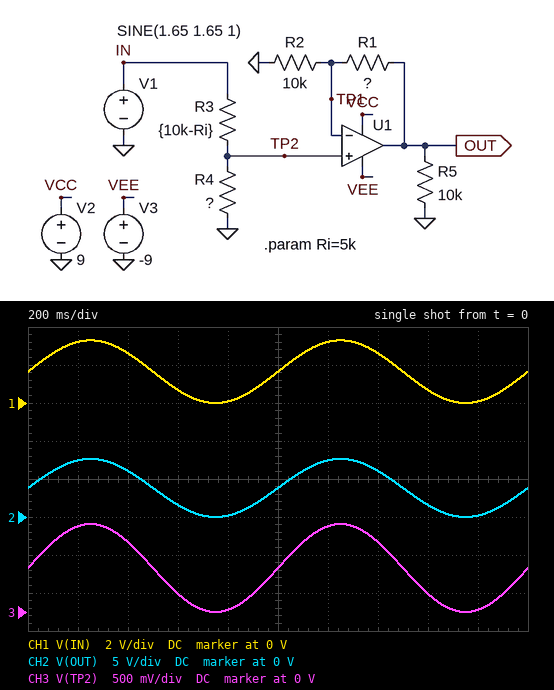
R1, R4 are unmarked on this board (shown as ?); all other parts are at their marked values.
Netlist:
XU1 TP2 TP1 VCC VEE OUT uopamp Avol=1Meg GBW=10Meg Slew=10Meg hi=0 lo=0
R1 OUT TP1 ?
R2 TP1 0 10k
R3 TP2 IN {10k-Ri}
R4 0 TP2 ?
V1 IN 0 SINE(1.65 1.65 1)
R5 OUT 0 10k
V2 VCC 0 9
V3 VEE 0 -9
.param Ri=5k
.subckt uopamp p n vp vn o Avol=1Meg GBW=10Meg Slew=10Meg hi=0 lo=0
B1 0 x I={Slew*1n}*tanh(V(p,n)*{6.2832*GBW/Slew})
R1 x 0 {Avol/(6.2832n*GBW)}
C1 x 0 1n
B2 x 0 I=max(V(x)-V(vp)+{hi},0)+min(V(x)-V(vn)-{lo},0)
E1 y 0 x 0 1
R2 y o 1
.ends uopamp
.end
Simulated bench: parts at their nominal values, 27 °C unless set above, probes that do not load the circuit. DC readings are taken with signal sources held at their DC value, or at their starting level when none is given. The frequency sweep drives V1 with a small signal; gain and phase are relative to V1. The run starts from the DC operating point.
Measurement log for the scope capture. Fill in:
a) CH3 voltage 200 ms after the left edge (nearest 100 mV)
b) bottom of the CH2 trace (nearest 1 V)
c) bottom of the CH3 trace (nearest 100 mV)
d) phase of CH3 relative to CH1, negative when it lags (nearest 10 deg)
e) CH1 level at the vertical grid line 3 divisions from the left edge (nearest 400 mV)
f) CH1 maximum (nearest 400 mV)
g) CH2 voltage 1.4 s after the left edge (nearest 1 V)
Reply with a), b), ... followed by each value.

a) 1.1 V
b) 0 V
c) 0 V
d) 0 deg
e) 800 mV
f) 3.2 V
g) 6 V
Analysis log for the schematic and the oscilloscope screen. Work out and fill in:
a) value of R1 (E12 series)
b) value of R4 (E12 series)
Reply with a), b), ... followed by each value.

a) 56 kΩ
b) 2.7 kΩ
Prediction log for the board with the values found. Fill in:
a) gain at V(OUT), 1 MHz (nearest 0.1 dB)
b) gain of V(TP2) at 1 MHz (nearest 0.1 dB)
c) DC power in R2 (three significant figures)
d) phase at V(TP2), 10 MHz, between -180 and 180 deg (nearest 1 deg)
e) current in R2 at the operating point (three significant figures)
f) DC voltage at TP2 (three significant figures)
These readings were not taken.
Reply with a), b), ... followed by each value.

a) 5.7 dB
b) -9.1 dB
c) 33.5 µW
d) 0 deg
e) 57.9 µA
f) 579 mV
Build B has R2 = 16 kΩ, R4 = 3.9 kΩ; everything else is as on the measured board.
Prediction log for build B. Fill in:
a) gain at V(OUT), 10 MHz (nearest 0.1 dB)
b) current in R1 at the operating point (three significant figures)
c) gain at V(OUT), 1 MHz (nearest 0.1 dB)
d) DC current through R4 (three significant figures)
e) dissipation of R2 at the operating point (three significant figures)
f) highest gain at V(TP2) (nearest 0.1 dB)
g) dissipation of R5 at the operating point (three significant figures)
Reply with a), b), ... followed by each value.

a) -7.4 dB
b) 45.2 µA
c) 5.1 dB
d) 185 µA
e) 32.7 µW
f) -7.2 dB
g) 1.06 mW
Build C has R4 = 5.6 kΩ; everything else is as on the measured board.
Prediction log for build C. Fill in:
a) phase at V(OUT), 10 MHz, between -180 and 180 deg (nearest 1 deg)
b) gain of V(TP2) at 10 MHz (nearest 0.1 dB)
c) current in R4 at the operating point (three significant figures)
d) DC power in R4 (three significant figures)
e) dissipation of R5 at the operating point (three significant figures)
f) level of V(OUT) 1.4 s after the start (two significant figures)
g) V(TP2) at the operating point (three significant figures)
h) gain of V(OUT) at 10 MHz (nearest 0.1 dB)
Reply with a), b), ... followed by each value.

a) -81 deg
b) -5.5 dB
c) 156 µA
d) 136 µW
e) 3.31 mW
f) 9.0 V
g) 872 mV
h) -5.6 dB
